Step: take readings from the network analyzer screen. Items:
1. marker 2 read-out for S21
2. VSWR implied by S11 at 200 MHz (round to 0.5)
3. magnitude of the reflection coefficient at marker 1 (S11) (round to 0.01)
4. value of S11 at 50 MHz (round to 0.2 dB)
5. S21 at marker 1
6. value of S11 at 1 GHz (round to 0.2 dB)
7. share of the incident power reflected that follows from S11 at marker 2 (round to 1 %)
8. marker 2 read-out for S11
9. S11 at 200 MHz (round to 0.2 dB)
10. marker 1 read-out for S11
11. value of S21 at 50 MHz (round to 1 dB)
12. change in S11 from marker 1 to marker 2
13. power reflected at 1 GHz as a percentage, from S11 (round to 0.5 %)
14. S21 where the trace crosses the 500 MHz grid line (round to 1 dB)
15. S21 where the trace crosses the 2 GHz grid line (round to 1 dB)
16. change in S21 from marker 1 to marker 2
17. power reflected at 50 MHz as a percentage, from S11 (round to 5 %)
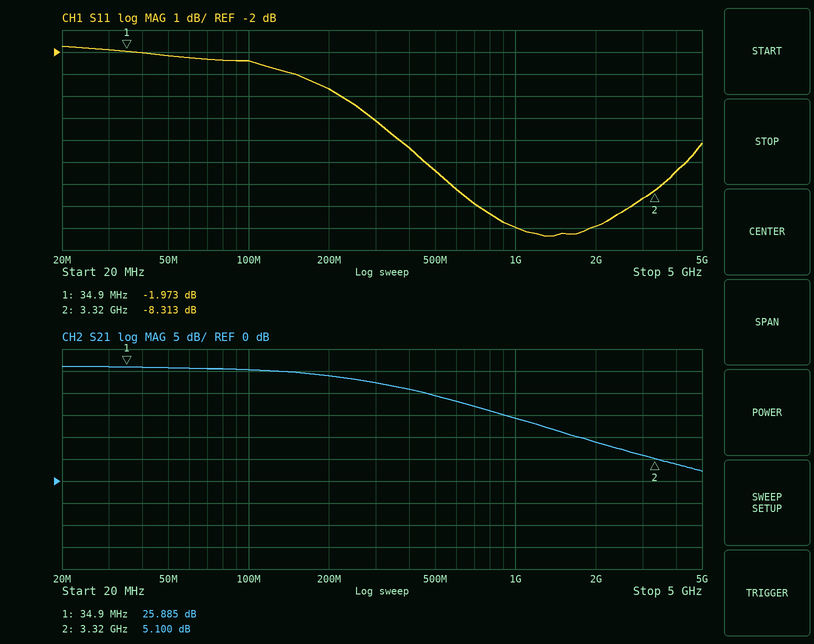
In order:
5.100 dB
5.0
0.80
-2.2 dB
25.885 dB
-10.0 dB
15 %
-8.313 dB
-3.6 dB
-1.973 dB
26 dB
-6.340 dB
10.0 %
19 dB
9 dB
-20.785 dB
60 %
